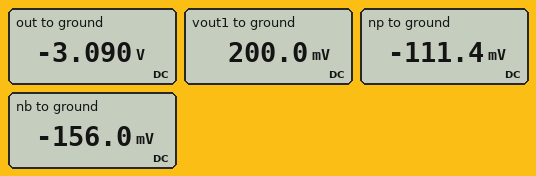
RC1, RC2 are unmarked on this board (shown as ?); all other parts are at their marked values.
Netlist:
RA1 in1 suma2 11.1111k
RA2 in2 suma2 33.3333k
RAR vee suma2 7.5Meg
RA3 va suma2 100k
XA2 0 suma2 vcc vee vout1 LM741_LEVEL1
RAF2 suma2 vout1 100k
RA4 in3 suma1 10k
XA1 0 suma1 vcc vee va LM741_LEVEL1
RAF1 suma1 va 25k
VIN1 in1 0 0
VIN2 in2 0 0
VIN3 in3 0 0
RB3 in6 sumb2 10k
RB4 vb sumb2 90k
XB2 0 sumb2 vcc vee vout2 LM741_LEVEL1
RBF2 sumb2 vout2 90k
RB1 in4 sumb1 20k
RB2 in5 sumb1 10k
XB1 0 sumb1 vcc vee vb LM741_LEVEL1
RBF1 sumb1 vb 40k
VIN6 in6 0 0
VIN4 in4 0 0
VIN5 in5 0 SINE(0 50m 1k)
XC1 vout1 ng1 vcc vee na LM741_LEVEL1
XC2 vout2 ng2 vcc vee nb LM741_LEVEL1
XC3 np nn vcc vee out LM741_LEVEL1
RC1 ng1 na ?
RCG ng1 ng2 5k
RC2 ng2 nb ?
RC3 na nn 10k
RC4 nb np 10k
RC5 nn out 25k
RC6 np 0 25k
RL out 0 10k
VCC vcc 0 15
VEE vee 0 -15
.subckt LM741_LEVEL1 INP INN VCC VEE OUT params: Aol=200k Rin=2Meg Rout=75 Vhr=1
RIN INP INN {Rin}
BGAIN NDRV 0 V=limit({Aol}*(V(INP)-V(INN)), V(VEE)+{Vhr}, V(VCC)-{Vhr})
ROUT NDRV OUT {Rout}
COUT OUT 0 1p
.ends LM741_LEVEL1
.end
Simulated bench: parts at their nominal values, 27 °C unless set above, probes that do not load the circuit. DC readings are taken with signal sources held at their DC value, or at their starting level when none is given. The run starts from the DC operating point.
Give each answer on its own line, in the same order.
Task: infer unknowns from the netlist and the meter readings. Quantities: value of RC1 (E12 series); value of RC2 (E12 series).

22 kΩ
3.9 kΩ
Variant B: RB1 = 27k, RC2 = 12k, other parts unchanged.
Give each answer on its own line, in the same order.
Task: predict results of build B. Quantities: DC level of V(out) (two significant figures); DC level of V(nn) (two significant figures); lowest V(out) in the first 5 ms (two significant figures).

-3.9 V
-340 mV
-7.8 V
